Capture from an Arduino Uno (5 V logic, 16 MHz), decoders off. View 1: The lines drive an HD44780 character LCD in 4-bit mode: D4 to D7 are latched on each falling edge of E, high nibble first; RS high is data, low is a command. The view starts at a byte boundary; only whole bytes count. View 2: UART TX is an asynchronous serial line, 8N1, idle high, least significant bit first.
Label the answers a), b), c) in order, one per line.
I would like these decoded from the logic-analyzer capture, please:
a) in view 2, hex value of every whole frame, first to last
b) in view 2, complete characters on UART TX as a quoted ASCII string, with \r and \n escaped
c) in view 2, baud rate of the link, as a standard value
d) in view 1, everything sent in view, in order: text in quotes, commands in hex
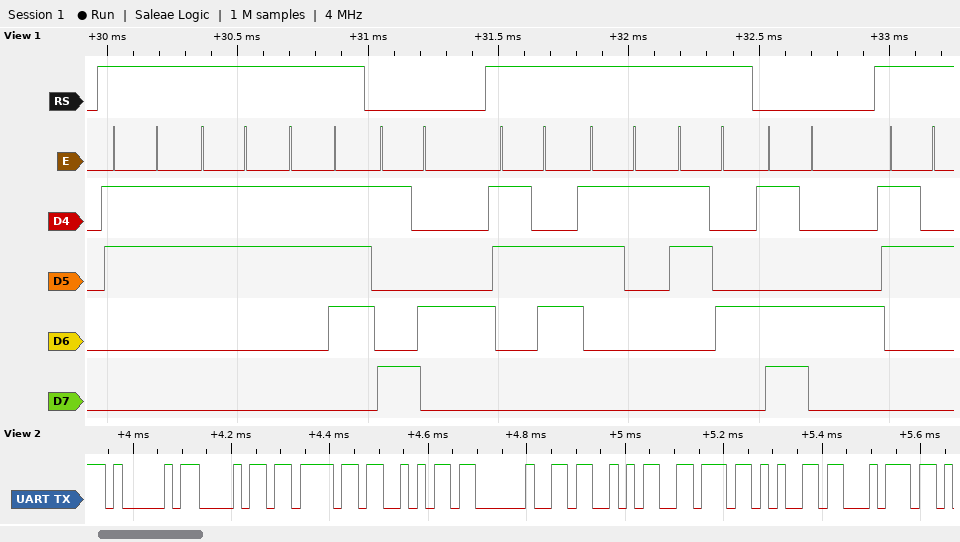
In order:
a) 41 68 6F 6A 20 53 76 65 74
b) "Ahoj Svet"
c) 57600 baud
d) "337" 0x94 "614" 0xD4 "2"
